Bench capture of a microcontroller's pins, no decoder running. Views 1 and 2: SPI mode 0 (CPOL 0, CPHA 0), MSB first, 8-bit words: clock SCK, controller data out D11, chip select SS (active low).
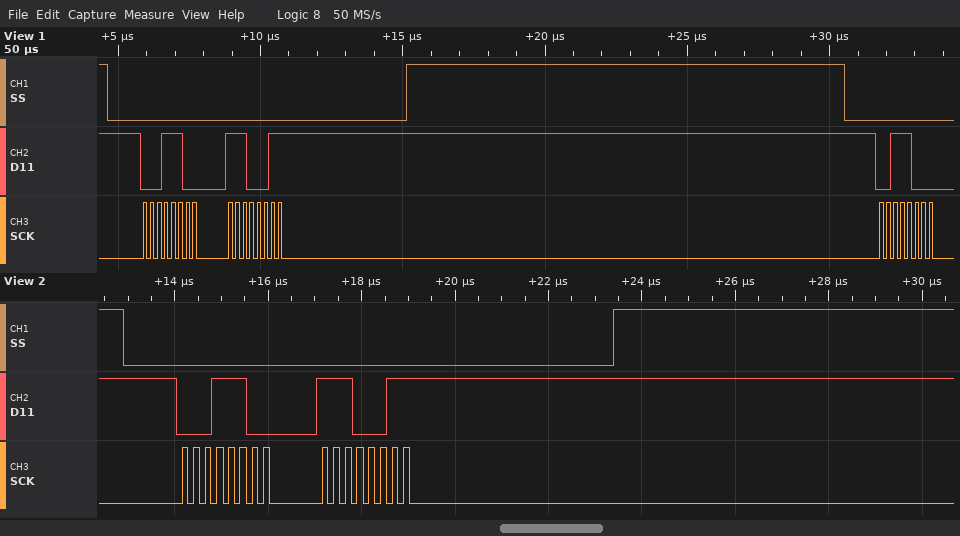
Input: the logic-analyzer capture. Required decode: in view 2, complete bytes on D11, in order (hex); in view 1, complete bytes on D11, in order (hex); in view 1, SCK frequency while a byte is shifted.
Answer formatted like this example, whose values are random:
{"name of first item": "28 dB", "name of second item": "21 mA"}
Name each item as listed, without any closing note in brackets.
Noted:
{"in view 2, complete bytes on D11, in order": "0x1C 0xE3", "in view 1, complete bytes on D11, in order": "1C E3 38", "in view 1, SCK frequency while a byte is shifted": "4 MHz"}
